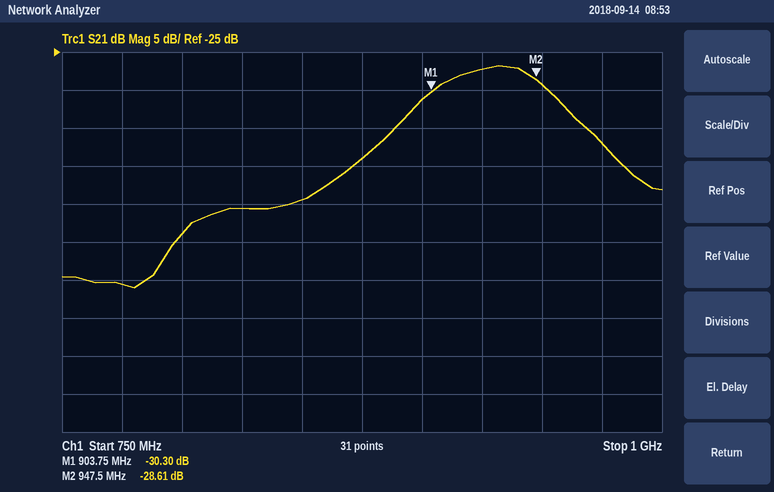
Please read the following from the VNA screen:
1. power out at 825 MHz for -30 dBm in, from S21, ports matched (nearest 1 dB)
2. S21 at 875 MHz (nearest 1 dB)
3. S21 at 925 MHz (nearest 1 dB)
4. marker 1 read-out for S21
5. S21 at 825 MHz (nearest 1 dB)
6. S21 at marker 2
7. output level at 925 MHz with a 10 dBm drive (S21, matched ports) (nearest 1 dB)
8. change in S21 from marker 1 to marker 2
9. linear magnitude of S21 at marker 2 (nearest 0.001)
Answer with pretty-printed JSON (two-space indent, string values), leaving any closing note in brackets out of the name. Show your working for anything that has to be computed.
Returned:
{
  "power out at 825 MHz for -30 dBm in, from S21, ports matched": "-30 dBm + (-46 dB) = -76 dBm",
  "S21 at 875 MHz": "-39 dB",
  "S21 at 925 MHz": "-27 dB",
  "marker 1 read-out for S21": "-30.30 dB",
  "S21 at 825 MHz": "-46 dB",
  "S21 at marker 2": "-28.61 dB",
  "output level at 925 MHz with a 10 dBm drive (S21, matched ports)": "10 dBm + (-27 dB) = -17 dBm",
  "change in S21 from marker 1 to marker 2": "-28.61 − (-30.3) = 1.69 dB",
  "linear magnitude of S21 at marker 2": "10^(-28.61/20) ≈ 0.037"
}
